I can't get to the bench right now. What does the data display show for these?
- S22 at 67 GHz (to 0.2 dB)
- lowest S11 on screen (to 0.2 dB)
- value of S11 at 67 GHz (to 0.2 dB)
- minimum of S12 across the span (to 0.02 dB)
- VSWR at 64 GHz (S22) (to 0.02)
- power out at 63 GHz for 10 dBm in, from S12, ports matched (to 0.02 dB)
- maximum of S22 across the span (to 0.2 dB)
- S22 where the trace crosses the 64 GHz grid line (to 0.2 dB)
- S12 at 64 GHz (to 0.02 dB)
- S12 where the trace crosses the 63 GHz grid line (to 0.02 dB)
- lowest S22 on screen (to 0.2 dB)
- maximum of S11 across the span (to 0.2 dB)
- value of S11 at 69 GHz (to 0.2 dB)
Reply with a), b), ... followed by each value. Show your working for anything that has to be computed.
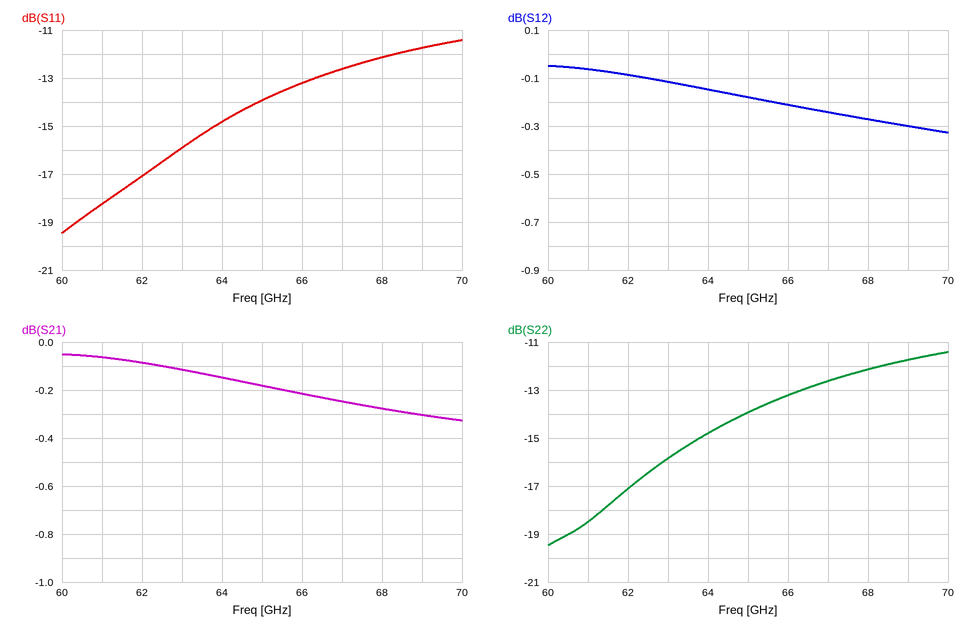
a) -12.6 dB
b) -19.4 dB
c) -12.6 dB
d) -0.32 dB
e) |Γ| = 10^(-14.8/20) = 0.1820; VSWR = (1 + 0.1820)/(1 − 0.1820) ≈ 1.44
f) 10 dBm + (-0.12 dB) = 9.88 dBm
g) -11.4 dB
h) -14.8 dB
i) -0.14 dB
j) -0.12 dB
k) -19.4 dB
l) -11.4 dB
m) -11.8 dB
